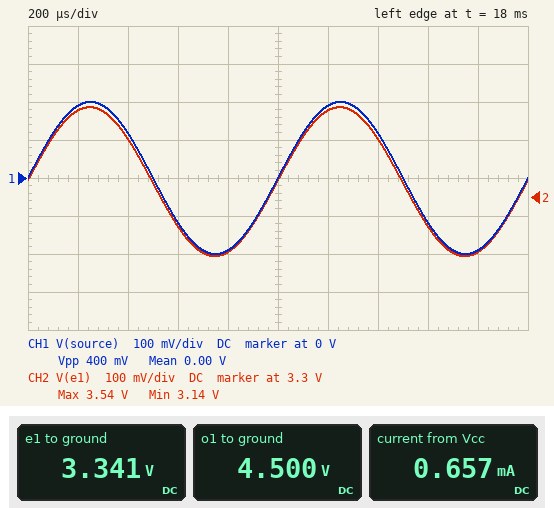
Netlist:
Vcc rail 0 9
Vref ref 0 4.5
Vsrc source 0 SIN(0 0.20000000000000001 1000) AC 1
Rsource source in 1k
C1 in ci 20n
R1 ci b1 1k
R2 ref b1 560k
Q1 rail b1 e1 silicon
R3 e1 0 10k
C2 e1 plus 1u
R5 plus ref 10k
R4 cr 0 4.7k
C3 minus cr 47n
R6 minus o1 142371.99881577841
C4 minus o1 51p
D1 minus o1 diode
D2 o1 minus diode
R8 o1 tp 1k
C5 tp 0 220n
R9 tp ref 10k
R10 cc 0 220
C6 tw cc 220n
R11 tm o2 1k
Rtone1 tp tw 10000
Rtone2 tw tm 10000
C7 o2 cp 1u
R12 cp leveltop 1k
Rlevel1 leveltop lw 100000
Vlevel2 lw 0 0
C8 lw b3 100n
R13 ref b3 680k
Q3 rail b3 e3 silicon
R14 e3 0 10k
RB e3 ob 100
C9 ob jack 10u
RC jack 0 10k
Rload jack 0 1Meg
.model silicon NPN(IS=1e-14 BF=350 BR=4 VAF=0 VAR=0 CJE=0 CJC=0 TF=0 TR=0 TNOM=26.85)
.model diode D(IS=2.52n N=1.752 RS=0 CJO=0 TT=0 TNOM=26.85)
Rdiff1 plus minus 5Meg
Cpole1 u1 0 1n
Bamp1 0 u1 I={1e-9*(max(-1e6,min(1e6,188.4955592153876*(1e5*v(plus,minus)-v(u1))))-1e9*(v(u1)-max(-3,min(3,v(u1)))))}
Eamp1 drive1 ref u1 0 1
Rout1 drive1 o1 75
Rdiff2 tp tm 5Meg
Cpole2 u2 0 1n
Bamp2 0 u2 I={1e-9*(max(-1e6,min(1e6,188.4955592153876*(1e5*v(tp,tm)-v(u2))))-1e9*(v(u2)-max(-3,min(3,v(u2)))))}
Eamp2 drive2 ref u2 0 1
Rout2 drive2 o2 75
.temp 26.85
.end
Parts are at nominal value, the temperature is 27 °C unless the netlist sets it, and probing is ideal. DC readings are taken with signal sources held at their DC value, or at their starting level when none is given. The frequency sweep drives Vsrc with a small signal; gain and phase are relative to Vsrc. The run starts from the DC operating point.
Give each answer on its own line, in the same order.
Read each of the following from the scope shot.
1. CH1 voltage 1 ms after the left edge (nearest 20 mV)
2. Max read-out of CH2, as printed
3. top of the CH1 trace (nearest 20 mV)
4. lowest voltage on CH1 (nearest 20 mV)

0 V
3.54 V
200 mV
-200 mV
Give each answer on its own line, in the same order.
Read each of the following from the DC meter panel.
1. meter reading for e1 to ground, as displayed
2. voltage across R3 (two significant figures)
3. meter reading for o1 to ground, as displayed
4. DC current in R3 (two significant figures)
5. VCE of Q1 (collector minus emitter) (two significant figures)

3.341 V
3.3 V
4.500 V
330 µA
5.7 V
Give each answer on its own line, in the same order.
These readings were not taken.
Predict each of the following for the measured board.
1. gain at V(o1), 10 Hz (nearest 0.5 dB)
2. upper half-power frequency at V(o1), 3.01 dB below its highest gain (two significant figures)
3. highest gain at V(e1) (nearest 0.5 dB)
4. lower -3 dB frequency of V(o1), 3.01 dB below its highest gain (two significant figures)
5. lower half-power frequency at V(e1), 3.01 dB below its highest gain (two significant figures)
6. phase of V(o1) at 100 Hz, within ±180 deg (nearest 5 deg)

-11.0 dB
19 kHz
0 dB
670 Hz
19 Hz
90 deg
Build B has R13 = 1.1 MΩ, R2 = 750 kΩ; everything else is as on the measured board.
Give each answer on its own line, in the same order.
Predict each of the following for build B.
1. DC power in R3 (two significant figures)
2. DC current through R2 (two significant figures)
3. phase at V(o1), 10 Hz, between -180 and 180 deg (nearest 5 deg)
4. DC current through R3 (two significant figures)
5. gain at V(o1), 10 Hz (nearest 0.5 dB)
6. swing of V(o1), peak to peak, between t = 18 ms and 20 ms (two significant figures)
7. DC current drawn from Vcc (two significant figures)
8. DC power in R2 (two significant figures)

1.0 mW
910 nA
130 deg
320 µA
-9.5 dB
1.2 V
610 µA
620 nW
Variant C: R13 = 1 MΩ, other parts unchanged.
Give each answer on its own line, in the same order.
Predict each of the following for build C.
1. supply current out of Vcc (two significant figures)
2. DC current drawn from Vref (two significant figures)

630 µA
1.8 µA
